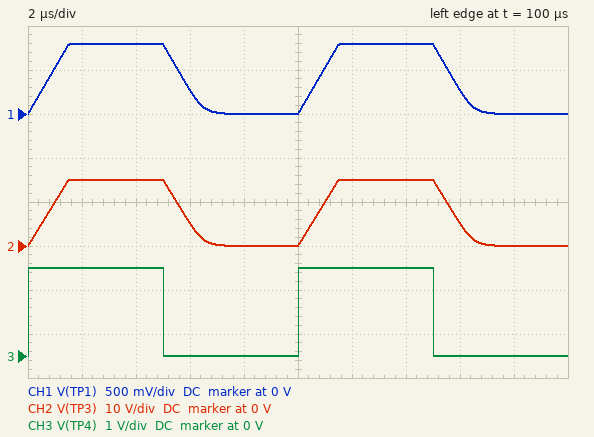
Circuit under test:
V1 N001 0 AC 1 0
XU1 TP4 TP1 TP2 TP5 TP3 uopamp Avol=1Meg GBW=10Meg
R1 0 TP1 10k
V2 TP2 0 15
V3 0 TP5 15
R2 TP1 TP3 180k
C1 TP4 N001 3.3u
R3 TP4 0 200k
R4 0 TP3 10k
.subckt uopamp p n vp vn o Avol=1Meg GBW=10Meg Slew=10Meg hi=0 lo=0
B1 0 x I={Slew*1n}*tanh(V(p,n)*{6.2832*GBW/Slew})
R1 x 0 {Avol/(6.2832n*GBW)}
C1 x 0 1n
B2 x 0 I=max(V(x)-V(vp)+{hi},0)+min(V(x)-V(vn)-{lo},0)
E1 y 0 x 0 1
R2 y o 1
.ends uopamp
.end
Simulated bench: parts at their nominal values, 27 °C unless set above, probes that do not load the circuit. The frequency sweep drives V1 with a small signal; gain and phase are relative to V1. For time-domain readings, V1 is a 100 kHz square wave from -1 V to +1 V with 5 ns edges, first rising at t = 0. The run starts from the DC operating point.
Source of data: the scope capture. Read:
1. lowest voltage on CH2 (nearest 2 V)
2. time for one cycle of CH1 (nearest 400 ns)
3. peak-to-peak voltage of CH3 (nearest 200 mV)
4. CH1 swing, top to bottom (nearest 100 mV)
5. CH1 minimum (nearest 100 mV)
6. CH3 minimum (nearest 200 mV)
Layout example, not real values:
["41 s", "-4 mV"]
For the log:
["0 V", "10.0 µs", "2.0 V", "800 mV", "0 V", "0 V"]
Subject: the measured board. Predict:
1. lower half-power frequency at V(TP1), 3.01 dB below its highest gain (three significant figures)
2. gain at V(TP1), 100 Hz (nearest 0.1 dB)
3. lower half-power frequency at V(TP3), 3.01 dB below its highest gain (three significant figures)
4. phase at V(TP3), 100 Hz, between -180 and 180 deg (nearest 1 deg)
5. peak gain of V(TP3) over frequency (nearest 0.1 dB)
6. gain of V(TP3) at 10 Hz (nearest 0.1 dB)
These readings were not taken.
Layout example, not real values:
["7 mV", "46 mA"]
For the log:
["241 mHz", "0 dB", "241 mHz", "0 deg", "25.6 dB", "25.6 dB"]
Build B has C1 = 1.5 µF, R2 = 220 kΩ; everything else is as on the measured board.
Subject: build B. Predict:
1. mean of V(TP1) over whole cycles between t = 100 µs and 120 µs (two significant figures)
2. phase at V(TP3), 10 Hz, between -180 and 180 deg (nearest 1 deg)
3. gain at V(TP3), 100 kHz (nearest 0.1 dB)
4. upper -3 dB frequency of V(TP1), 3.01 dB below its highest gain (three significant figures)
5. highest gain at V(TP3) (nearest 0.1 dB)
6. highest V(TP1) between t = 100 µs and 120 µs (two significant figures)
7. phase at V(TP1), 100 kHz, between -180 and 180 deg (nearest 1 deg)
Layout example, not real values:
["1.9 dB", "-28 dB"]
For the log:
["330 mV", "3 deg", "27.0 dB", "435 kHz", "27.2 dB", "650 mV", "-13 deg"]
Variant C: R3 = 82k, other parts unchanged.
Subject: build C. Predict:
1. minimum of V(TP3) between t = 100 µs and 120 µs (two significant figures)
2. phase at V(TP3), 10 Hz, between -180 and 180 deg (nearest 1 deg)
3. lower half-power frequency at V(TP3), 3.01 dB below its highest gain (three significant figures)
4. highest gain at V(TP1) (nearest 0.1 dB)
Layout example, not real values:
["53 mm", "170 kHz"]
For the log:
["-8.4 mV", "3 deg", "588 mHz", "0 dB"]
